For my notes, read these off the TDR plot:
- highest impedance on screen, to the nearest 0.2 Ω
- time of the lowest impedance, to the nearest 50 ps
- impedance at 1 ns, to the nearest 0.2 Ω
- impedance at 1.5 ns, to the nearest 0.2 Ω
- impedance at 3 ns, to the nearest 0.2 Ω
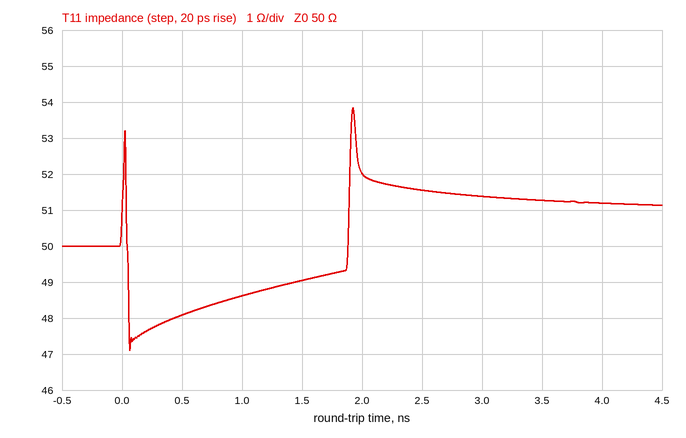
53.8 Ω
50 ps
48.6 Ω
49.0 Ω
51.4 Ω
